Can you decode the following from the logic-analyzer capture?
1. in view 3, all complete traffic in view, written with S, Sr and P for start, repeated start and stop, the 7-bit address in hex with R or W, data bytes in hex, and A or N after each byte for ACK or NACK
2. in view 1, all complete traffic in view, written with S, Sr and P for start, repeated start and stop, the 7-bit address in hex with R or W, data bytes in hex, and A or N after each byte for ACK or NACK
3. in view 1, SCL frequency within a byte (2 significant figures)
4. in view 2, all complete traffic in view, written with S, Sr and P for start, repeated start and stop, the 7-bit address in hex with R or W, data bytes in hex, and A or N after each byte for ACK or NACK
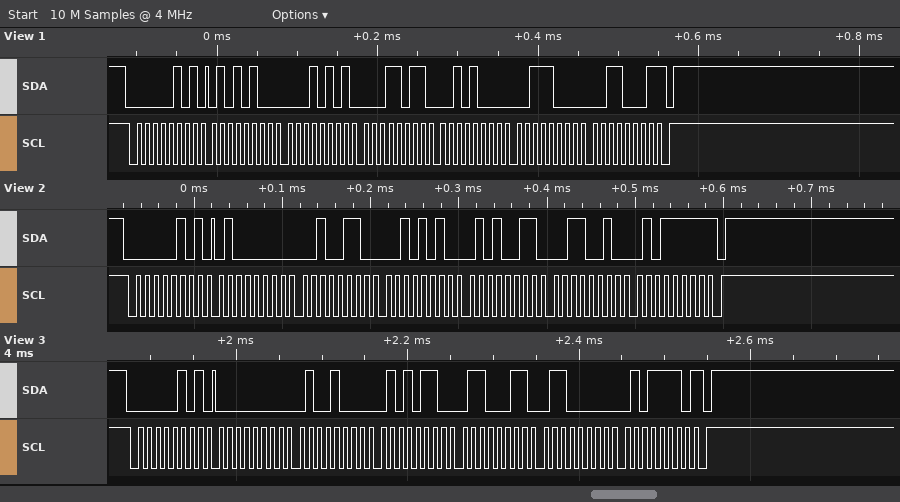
S 02R A 00 A 48 A 56 A 63 A 60 A 5E N P
S 02R A 54 A 15 A 1B A 28 A 38 A 31 N P
100 kHz
S 02R A 40 A 26 A 2A A 53 A 32 A 5F N P
